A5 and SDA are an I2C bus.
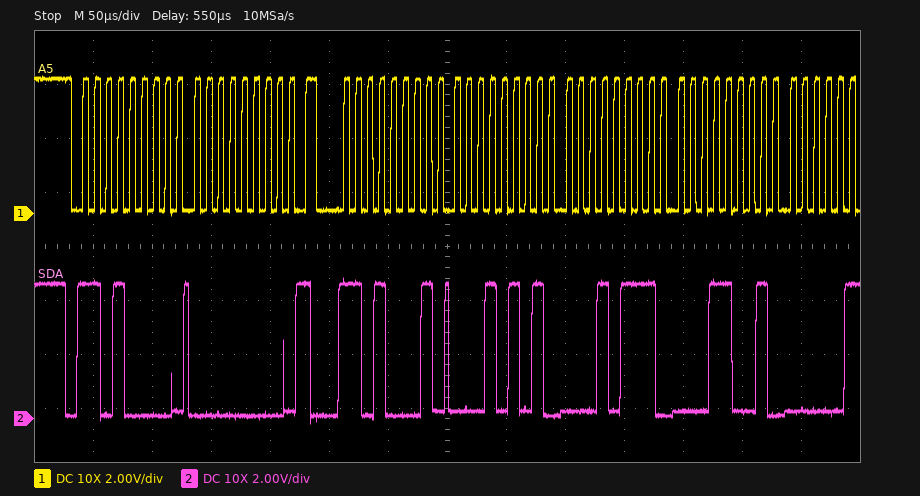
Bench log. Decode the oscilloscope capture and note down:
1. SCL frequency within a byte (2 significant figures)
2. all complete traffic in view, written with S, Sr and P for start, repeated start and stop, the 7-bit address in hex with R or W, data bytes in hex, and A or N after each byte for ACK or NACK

100 kHz
S 68W A 00 A Sr 68R A 15 A 17 A 19 A
